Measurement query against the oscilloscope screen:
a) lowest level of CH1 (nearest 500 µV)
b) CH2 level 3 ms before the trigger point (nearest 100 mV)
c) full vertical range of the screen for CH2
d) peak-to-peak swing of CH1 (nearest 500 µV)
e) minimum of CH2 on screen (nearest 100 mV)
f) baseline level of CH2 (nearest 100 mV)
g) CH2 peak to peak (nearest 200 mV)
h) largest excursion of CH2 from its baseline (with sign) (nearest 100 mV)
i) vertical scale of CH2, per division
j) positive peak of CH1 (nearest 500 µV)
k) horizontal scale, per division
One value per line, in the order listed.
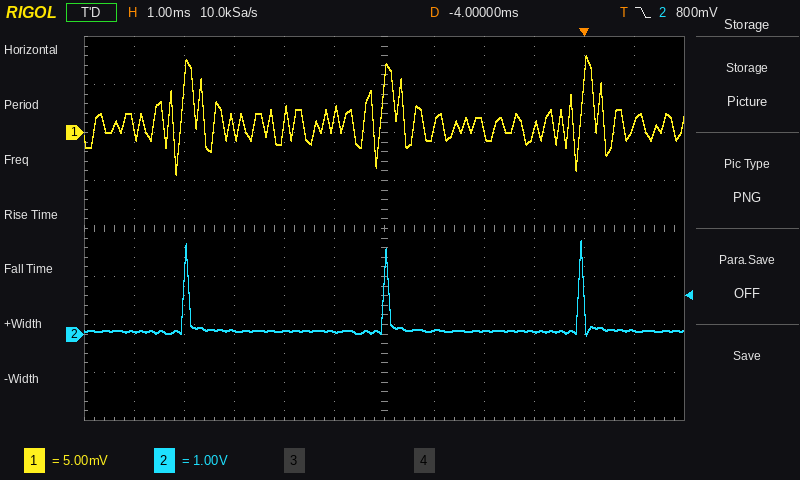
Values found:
-4.5 mV
100 mV
8 V
12.5 mV
0.0 V
100 mV
2.0 V
+1.9 V
1 V
8.0 mV
1 ms
